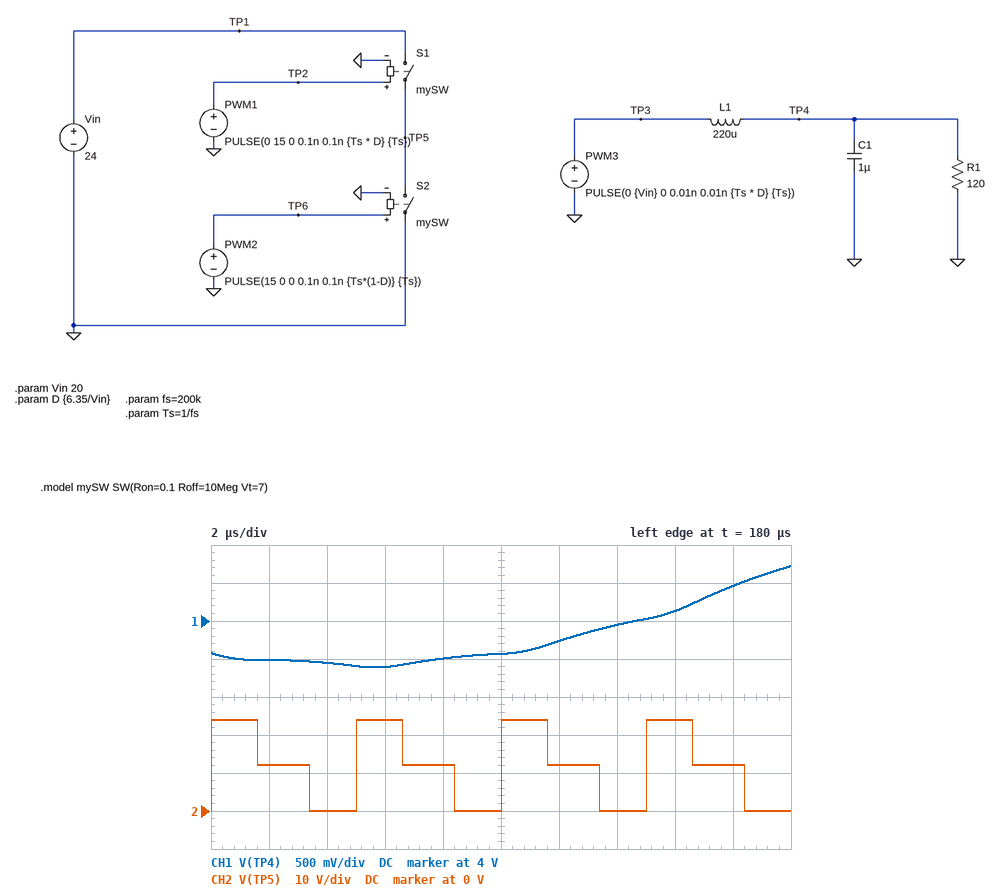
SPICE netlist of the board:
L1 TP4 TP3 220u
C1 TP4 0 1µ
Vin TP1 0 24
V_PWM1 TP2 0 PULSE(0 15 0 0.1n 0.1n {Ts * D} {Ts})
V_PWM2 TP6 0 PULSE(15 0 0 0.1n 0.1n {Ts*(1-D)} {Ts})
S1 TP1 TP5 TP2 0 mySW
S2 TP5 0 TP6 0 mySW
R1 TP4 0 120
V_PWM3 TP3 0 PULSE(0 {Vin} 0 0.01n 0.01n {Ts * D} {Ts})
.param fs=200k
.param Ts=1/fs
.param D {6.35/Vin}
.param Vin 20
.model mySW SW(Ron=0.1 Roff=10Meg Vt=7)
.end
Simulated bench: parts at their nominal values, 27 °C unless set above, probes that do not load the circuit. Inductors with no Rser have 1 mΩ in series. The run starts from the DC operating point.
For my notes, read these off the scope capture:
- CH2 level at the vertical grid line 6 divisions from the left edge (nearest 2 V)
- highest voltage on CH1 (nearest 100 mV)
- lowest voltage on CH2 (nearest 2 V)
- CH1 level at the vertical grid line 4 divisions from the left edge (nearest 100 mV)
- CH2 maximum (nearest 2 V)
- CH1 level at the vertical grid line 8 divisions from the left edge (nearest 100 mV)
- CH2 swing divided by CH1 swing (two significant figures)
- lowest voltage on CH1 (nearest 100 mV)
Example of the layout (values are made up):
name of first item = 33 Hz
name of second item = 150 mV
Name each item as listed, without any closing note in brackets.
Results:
CH2 level at the vertical grid line 6 divisions from the left edge = 12 V
highest voltage on CH1 = 4.7 V
lowest voltage on CH2 = 0 V
CH1 level at the vertical grid line 4 divisions from the left edge = 3.5 V
CH2 maximum = 24 V
CH1 level at the vertical grid line 8 divisions from the left edge = 4.1 V
CH2 swing divided by CH1 swing = 18
lowest voltage on CH1 = 3.4 V
